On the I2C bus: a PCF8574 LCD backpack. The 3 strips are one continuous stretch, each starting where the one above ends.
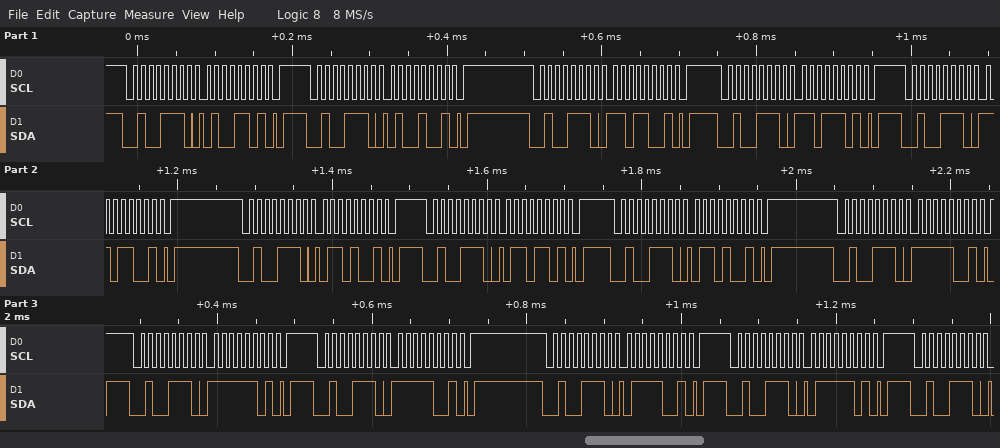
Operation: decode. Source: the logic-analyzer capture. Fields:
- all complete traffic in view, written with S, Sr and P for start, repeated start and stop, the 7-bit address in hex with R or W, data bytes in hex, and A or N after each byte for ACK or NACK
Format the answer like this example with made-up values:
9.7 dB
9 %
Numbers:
S 27W A 4D A P S 27W A 49 A P S 27W A D9 A P S 27W A DD A P S 27W A D9 A P S 27W A 69 A P S 27W A 6D A P S 27W A 69 A P S 27W A F9 A P S 27W A FD A P S 27W A F9 A P S 27W A 79 A P S 27W A 7D A P S 27W A
